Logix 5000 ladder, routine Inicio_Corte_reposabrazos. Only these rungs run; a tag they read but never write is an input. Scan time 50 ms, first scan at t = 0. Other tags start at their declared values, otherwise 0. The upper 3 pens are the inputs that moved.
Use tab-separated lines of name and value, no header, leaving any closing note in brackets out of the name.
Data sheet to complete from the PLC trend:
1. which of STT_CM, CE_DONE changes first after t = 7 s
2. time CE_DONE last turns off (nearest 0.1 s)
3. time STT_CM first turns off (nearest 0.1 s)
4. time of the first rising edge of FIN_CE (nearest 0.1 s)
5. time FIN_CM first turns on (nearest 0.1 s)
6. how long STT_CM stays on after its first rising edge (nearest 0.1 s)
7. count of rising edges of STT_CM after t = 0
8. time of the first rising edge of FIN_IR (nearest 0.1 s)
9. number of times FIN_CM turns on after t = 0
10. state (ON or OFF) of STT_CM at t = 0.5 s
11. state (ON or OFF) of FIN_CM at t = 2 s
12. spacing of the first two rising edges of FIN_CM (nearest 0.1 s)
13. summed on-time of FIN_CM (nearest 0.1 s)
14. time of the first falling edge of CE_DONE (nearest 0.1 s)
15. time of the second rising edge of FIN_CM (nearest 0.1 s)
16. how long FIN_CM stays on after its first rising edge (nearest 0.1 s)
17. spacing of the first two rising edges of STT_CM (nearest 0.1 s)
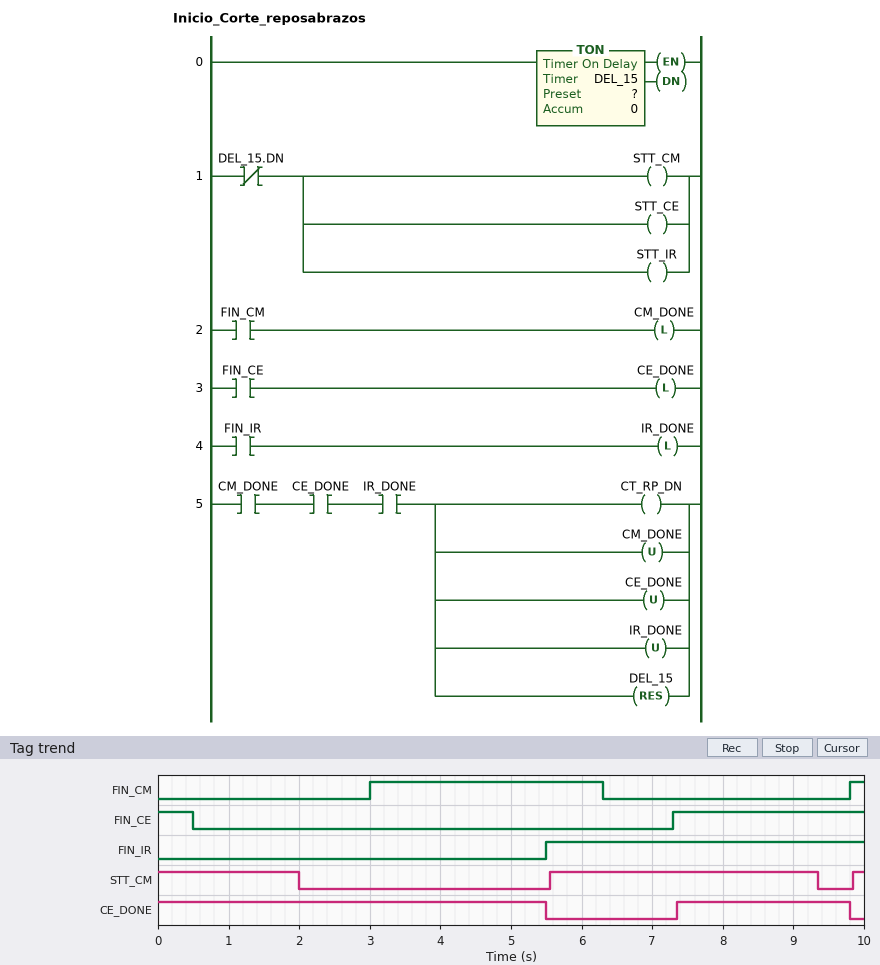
which of STT_CM, CE_DONE changes first after t = 7 s	CE_DONE
time CE_DONE last turns off	9.8 s
time STT_CM first turns off	2.0 s
time of the first rising edge of FIN_CE	7.3 s
time FIN_CM first turns on	3.0 s
how long STT_CM stays on after its first rising edge	3.8 s
count of rising edges of STT_CM after t = 0	2
time of the first rising edge of FIN_IR	5.5 s
number of times FIN_CM turns on after t = 0	2
state (ON or OFF) of STT_CM at t = 0.5 s	ON
state (ON or OFF) of FIN_CM at t = 2 s	OFF
spacing of the first two rising edges of FIN_CM	6.8 s
summed on-time of FIN_CM	3.5 s
time of the first falling edge of CE_DONE	5.5 s
time of the second rising edge of FIN_CM	9.8 s
how long FIN_CM stays on after its first rising edge	3.3 s
spacing of the first two rising edges of STT_CM	4.3 s
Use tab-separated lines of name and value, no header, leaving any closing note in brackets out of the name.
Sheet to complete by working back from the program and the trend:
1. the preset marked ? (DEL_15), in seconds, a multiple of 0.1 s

the preset marked ? (DEL_15), in seconds, a multiple of 0.1 s	2.0 s
